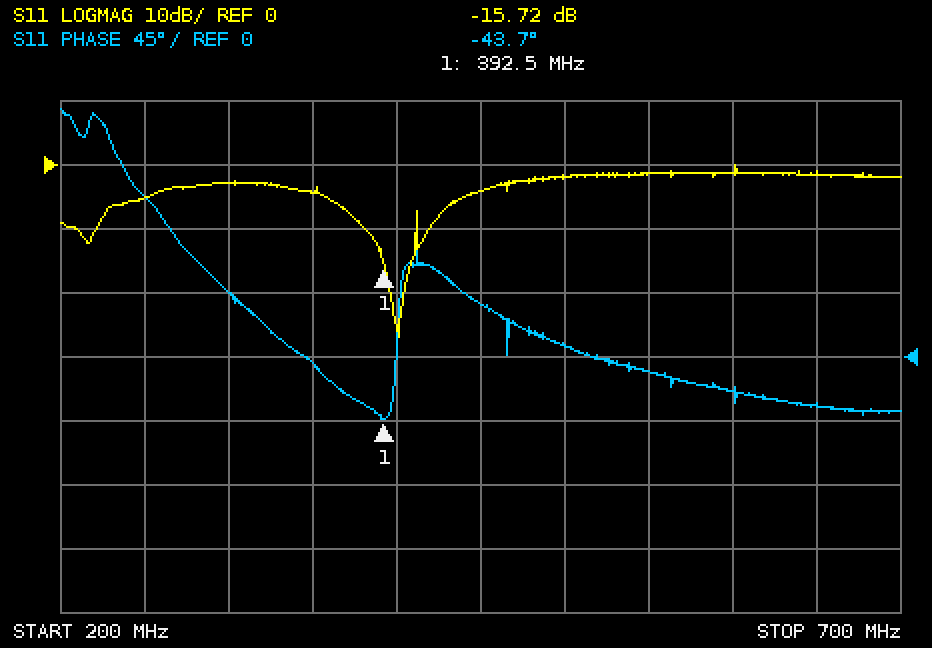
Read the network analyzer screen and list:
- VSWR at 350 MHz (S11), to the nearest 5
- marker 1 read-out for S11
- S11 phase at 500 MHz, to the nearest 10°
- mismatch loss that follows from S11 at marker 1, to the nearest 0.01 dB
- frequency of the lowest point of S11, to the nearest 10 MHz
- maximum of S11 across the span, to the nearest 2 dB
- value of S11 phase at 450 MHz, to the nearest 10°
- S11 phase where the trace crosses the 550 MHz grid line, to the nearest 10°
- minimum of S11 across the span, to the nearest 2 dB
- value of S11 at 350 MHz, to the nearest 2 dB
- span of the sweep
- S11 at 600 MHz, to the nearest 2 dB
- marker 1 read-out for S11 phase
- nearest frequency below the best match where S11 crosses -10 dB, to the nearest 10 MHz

5
-15.72 dB
10°
0.12 dB
400 MHz
0 dB
40°
-10°
-26 dB
-4 dB
500 MHz
-2 dB
-43.7°
380 MHz
